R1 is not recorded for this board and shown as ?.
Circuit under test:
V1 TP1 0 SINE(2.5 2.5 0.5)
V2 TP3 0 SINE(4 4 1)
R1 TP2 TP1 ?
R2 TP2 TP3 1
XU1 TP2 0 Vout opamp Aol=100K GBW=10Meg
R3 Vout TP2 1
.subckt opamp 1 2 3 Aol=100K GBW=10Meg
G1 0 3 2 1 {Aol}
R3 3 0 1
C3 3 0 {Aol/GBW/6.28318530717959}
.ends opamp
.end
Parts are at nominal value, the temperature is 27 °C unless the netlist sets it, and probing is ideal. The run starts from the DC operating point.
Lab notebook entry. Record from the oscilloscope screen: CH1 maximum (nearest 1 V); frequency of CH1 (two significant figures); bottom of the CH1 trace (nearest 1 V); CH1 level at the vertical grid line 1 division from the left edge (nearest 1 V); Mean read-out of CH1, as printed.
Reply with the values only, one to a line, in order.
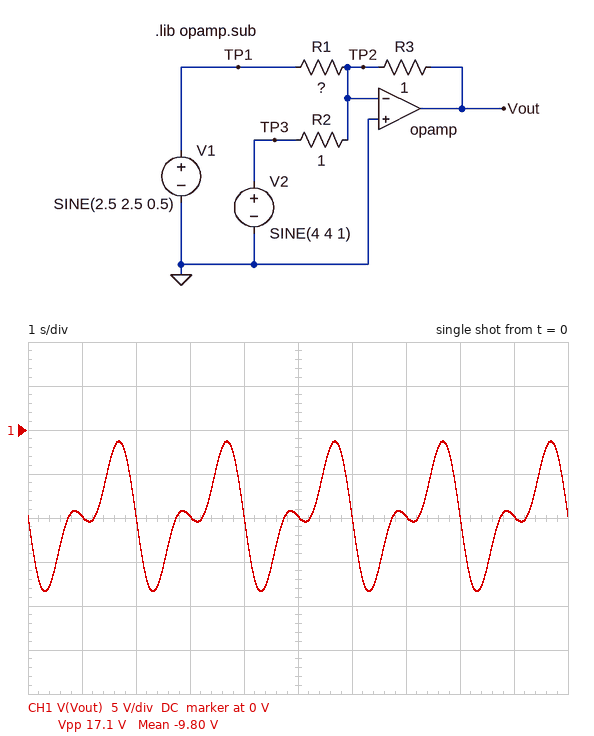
-1 V
500 mHz
-18 V
-10 V
-9.80 V
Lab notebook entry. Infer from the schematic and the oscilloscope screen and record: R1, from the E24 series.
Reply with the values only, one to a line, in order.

0.43 Ω
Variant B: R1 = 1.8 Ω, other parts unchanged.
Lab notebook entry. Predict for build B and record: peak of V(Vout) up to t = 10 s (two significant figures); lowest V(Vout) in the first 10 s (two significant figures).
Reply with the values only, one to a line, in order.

-380 mV
-10 V
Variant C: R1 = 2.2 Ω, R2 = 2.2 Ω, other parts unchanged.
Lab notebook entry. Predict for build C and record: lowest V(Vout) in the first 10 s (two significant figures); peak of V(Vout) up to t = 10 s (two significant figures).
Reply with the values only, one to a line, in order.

-5.6 V
-290 mV
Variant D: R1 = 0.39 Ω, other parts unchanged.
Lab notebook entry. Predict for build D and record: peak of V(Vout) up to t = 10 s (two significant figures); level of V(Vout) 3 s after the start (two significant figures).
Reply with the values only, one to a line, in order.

-1.4 V
-10 V
